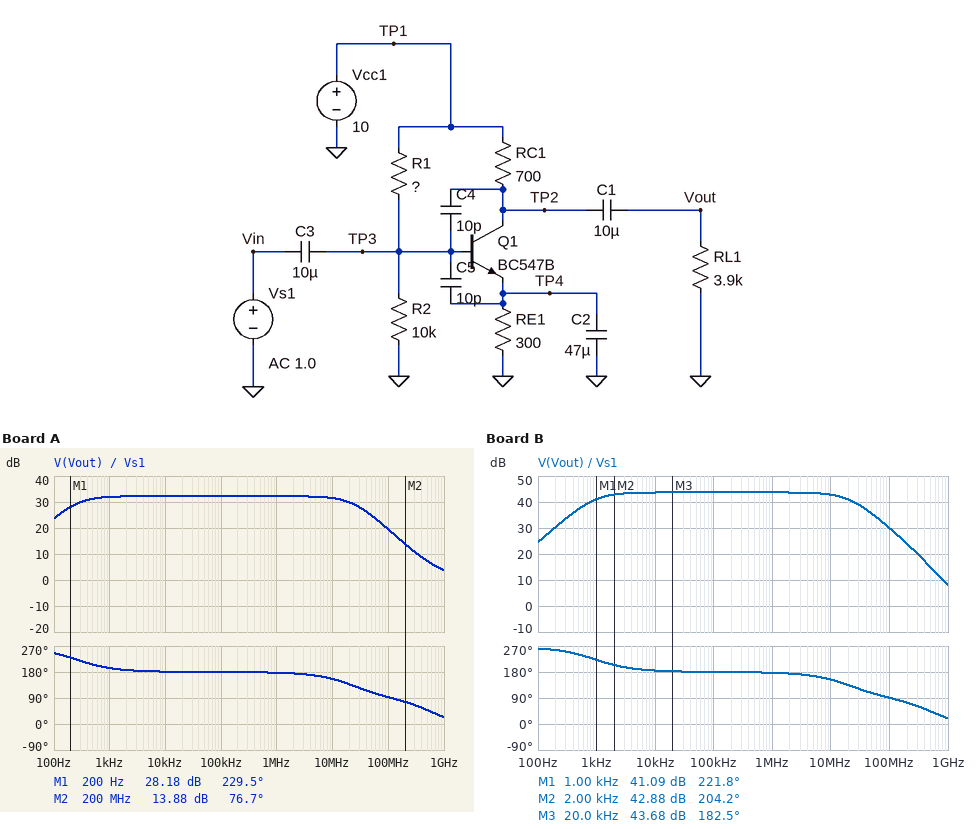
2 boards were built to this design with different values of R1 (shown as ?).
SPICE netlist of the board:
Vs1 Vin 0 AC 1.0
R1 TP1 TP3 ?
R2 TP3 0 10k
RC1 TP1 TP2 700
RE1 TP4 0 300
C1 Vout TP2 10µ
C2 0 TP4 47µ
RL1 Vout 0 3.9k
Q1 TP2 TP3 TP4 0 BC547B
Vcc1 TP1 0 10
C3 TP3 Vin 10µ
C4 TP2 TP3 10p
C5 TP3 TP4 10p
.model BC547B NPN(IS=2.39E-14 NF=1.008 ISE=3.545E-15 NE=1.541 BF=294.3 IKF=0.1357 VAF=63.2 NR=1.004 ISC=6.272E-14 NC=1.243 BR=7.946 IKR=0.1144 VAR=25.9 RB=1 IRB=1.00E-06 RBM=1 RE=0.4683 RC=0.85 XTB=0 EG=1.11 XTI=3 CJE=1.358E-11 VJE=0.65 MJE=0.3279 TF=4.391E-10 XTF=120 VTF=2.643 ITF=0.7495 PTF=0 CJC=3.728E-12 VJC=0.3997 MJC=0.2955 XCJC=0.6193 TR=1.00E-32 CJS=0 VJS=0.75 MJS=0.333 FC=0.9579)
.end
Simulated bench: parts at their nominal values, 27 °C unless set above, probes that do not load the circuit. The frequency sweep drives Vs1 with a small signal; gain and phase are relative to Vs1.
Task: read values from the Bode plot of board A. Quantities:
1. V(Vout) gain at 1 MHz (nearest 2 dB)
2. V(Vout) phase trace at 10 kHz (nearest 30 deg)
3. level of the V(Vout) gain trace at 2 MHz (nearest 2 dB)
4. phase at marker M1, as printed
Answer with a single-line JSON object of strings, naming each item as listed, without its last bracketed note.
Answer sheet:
{"V(Vout) gain at 1 MHz": "32 dB", "V(Vout) phase trace at 10 kHz": "180 deg", "level of the V(Vout) gain trace at 2 MHz": "32 dB", "phase at marker M1, as printed": "229.5 deg"}
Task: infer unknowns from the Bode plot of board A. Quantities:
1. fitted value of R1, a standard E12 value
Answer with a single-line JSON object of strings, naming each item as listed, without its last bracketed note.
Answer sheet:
{"fitted value of R1, a standard E12 value": "68 kΩ"}
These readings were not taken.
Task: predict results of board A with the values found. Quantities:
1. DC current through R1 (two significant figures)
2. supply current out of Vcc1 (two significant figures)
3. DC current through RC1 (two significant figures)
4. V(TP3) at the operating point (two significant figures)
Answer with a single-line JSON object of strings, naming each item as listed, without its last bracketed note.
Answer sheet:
{"DC current through R1": "130 µA", "supply current out of Vcc1": "2.0 mA", "DC current through RC1": "1.9 mA", "V(TP3) at the operating point": "1.2 V"}
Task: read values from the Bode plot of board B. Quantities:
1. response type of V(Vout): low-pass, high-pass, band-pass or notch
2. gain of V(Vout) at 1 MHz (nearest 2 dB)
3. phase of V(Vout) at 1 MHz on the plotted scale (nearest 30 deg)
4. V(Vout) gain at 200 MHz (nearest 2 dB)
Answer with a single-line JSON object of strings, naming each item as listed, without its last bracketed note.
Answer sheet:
{"response type of V(Vout): low-pass, high-pass, band-pass or notch": "band-pass", "gain of V(Vout) at 1 MHz": "44 dB", "phase of V(Vout) at 1 MHz on the plotted scale": "180 deg", "V(Vout) gain at 200 MHz": "24 dB"}
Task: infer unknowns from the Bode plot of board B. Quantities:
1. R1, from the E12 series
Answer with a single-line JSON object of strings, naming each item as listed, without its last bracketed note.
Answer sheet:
{"R1, from the E12 series": "18 kΩ"}
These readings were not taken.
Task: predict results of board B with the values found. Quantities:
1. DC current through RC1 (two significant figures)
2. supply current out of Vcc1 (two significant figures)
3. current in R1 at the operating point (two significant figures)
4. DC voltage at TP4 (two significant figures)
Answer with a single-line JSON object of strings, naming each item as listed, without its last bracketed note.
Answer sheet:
{"DC current through RC1": "8.8 mA", "supply current out of Vcc1": "9.2 mA", "current in R1 at the operating point": "370 µA", "DC voltage at TP4": "2.7 V"}
